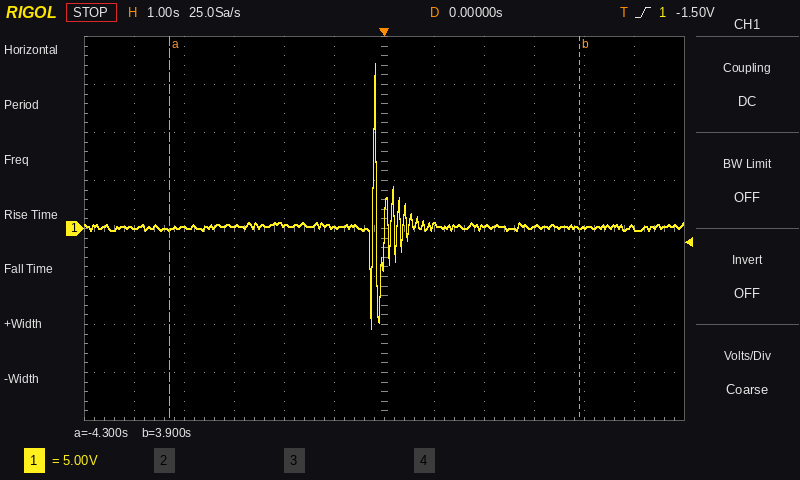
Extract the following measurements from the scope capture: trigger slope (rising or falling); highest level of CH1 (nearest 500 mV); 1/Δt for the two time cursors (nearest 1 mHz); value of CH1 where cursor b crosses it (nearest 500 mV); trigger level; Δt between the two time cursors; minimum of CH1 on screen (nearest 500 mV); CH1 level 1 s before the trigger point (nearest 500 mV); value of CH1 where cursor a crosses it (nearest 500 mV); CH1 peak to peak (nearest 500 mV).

rising
17.0 V
122 mHz
0.0 V
-1.50 V
8.2 s
-10.5 V
0.0 V
0.0 V
27.5 V
